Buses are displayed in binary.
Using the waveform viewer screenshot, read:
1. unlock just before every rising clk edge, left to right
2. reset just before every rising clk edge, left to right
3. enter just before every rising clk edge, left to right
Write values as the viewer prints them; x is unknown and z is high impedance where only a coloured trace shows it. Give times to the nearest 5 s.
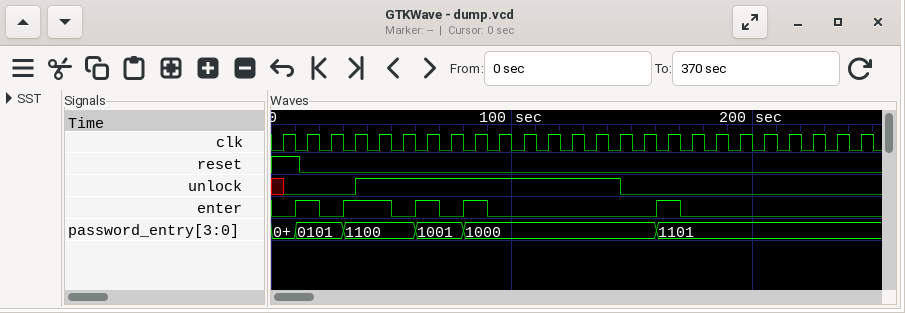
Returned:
x 0 0 0 1 1 1 1 1 1 1 1 1 1 1 0 0 0 0 0 0 0 0 0 0
1 0 0 0 0 0 0 0 0 0 0 0 0 0 0 0 0 0 0 0 0 0 0 0 0
0 1 0 1 1 0 1 0 1 0 0 0 0 0 0 0 1 0 0 0 0 0 0 0 0
